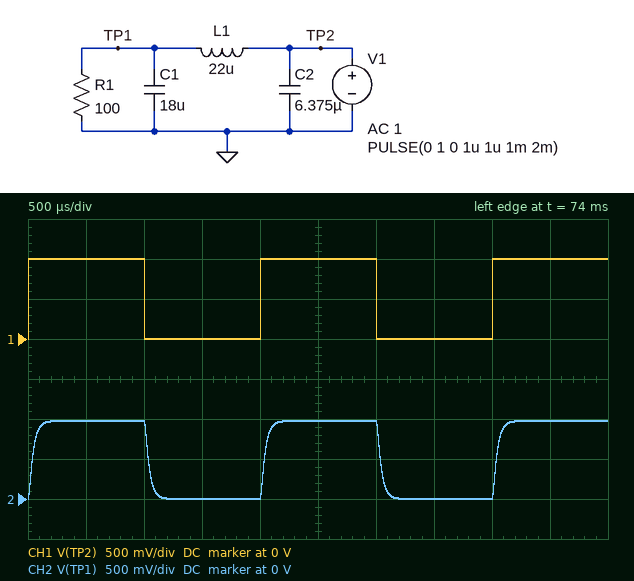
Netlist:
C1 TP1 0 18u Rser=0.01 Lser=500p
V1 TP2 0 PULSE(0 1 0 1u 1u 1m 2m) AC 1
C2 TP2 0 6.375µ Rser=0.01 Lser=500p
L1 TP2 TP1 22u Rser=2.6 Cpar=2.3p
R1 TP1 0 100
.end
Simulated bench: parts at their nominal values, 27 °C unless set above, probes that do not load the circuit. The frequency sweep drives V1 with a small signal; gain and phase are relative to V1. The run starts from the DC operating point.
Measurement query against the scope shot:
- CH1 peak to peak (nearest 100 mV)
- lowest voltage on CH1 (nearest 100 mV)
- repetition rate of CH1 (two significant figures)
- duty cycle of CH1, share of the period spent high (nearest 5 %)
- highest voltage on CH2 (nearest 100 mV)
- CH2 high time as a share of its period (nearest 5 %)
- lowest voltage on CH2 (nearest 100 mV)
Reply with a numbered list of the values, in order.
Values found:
1. 1.0 V
2. 0 V
3. 500 Hz
4. 50 %
5. 1.0 V
6. 50 %
7. 0 V
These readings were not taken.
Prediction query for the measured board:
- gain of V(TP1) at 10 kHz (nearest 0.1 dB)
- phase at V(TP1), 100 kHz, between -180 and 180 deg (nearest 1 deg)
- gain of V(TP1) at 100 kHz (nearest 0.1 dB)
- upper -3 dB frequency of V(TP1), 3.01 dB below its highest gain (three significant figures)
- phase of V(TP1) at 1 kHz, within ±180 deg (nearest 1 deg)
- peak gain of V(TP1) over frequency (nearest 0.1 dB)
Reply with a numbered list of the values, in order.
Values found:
1. -9.6 dB
2. -163 deg
3. -44.0 dB
4. 4.18 kHz
5. -16 deg
6. -0.2 dB
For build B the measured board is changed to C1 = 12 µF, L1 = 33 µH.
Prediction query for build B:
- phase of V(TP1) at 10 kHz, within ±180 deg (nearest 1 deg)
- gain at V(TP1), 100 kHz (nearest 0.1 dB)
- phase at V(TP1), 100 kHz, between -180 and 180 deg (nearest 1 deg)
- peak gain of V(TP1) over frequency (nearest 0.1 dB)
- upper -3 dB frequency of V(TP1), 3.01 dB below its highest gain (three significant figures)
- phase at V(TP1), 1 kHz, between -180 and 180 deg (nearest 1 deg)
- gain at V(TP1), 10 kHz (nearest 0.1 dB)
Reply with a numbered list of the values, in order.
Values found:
1. -105 deg
2. -43.9 dB
3. -168 deg
4. -0.2 dB
5. 7.22 kHz
6. -11 deg
7. -6.3 dB
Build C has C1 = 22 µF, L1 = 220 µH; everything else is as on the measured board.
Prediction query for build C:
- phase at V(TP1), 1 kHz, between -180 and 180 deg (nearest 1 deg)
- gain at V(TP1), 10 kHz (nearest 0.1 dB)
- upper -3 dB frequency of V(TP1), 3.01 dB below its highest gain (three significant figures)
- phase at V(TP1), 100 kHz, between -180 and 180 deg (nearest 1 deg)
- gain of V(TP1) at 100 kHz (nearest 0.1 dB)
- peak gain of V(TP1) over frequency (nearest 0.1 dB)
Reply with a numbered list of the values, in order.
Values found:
1. -24 deg
2. -25.3 dB
3. 2.75 kHz
4. -171 deg
5. -65.6 dB
6. 2.1 dB
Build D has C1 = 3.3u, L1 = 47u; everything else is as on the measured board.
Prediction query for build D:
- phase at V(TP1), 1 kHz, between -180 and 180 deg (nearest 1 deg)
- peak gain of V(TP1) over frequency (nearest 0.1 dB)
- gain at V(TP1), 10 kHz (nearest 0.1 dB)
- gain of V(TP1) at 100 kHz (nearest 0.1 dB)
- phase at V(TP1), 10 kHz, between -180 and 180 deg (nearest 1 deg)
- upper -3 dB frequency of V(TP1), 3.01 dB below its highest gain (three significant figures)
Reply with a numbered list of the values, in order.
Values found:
1. -3 deg
2. 3.2 dB
3. 3.0 dB
4. -35.6 dB
5. -54 deg
6. 15.4 kHz
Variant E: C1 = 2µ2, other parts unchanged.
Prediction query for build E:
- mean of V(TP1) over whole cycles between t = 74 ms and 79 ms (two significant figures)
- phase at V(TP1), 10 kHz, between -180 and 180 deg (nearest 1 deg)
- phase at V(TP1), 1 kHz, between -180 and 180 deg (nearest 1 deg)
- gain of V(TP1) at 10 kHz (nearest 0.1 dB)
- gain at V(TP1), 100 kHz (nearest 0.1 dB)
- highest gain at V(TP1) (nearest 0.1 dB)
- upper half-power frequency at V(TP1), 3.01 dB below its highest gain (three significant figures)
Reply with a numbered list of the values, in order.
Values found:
1. 490 mV
2. -24 deg
3. -2 deg
4. 0.8 dB
5. -25.3 dB
6. 2.1 dB
7. 27.5 kHz
